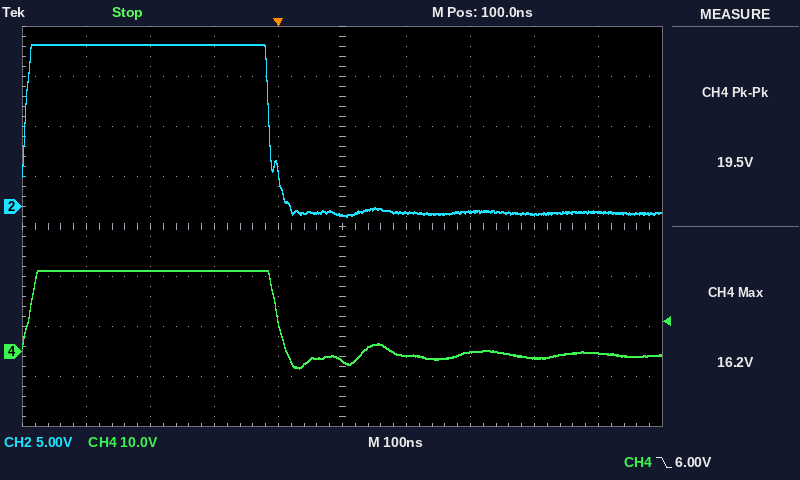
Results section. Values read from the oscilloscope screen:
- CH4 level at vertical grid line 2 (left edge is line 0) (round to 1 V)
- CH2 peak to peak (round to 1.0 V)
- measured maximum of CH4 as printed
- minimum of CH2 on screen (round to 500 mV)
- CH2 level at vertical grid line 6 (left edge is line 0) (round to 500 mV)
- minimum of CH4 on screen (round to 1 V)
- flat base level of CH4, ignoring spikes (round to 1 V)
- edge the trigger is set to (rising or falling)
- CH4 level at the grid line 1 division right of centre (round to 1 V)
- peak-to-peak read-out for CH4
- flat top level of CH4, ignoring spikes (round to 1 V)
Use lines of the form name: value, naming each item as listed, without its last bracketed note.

CH4 level at vertical grid line 2 (left edge is line 0): 16 V
CH2 peak to peak: 17.0 V
measured maximum of CH4 as printed: 16.2 V
minimum of CH2 on screen: -1.0 V
CH2 level at vertical grid line 6 (left edge is line 0): -500 mV
minimum of CH4 on screen: -3 V
flat base level of CH4, ignoring spikes: -1 V
edge the trigger is set to: falling
CH4 level at the grid line 1 division right of centre: -1 V
peak-to-peak read-out for CH4: 19.5 V
flat top level of CH4, ignoring spikes: 16 V
